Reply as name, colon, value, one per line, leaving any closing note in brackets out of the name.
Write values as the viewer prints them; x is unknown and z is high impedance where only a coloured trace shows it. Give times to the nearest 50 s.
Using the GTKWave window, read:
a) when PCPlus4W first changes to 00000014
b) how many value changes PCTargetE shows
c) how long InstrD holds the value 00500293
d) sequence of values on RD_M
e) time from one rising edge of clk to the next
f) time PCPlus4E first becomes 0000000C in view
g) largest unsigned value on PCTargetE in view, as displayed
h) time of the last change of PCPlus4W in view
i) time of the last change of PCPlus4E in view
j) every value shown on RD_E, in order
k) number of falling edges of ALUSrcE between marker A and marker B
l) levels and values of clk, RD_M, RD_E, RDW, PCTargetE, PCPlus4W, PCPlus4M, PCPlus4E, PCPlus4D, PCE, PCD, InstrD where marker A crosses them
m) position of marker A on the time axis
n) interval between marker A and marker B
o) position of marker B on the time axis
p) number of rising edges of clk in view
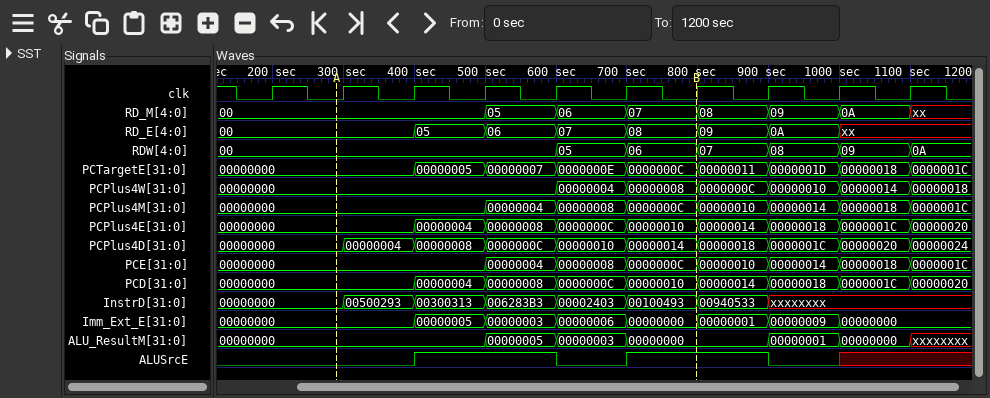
when PCPlus4W first changes to 00000014: 1000 s
how many value changes PCTargetE shows: 8
how long InstrD holds the value 00500293: 100 s
sequence of values on RD_M: 00, 05, 06, 07, 08, 09, 0A, xx
time from one rising edge of clk to the next: 100 s
time PCPlus4E first becomes 0000000C in view: 600 s
largest unsigned value on PCTargetE in view, as displayed: 0000001D
time of the last change of PCPlus4W in view: 1100 s
time of the last change of PCPlus4E in view: 1100 s
every value shown on RD_E, in order: 00, 05, 06, 07, 08, 09, 0A, xx
number of falling edges of ALUSrcE between marker A and marker B: 1
levels and values of clk, RD_M, RD_E, RDW, PCTargetE, PCPlus4W, PCPlus4M, PCPlus4E, PCPlus4D, PCE, PCD, InstrD where marker A crosses them: clk=0, RD_M=00, RD_E=00, RDW=00, PCTargetE=00000000, PCPlus4W=00000000, PCPlus4M=00000000, PCPlus4E=00000000, PCPlus4D=00000000, PCE=00000000, PCD=00000000, InstrD=00000000
position of marker A on the time axis: 300 s
interval between marker A and marker B: 500 s
position of marker B on the time axis: 800 s
number of rising edges of clk in view: 10
